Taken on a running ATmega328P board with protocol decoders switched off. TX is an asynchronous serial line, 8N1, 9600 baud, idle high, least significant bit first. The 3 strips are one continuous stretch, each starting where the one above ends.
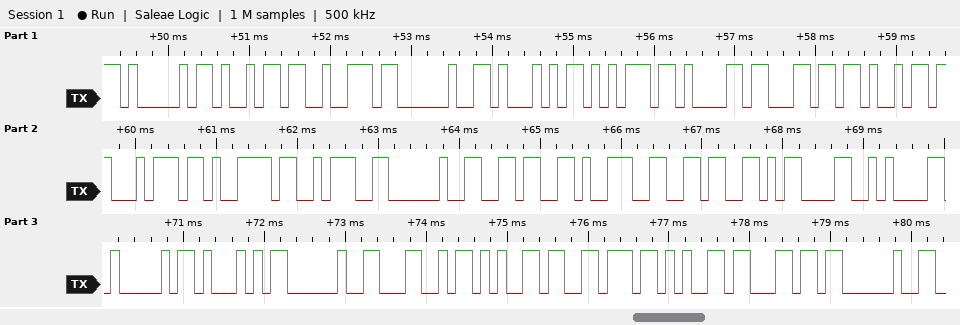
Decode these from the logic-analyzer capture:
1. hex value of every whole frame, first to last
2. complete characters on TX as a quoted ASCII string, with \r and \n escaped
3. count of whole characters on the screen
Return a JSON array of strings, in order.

["41 69 72 20 51 75 61 6C 69 74 79 3A 20 36 39 36 0D 0A 41 51 20 4C 65 76 65 6C 20", "\"Air Quality: 696\\r\\nAQ Level \"", "27"]
